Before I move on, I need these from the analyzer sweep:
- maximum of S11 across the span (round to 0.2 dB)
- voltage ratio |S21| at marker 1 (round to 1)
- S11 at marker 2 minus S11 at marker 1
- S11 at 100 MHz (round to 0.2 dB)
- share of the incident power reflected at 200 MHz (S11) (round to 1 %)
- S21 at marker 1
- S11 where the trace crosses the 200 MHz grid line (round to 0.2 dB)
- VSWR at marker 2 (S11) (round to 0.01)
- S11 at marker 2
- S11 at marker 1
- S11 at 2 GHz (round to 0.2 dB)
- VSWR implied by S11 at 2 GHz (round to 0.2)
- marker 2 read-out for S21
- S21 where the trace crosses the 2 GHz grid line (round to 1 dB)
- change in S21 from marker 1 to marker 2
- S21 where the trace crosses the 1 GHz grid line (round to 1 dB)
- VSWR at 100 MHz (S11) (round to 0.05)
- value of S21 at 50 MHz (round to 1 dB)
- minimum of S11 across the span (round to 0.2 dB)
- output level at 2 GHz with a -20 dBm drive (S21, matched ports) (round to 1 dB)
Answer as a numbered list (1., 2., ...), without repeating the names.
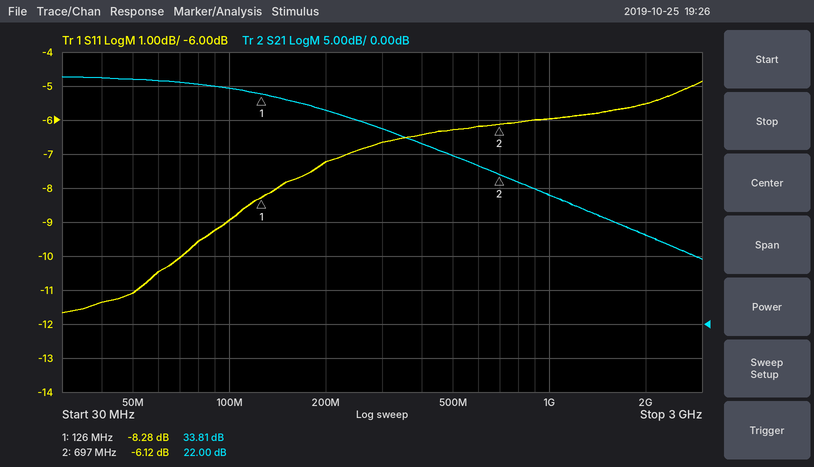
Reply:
1. -4.8 dB
2. 49
3. 2.16 dB
4. -9.0 dB
5. 19 %
6. 33.81 dB
7. -7.2 dB
8. 2.95
9. -6.12 dB
10. -8.28 dB
11. -5.6 dB
12. 3.2
13. 22.00 dB
14. 13 dB
15. -11.81 dB
16. 19 dB
17. 2.10
18. 36 dB
19. -11.6 dB
20. -7 dBm
